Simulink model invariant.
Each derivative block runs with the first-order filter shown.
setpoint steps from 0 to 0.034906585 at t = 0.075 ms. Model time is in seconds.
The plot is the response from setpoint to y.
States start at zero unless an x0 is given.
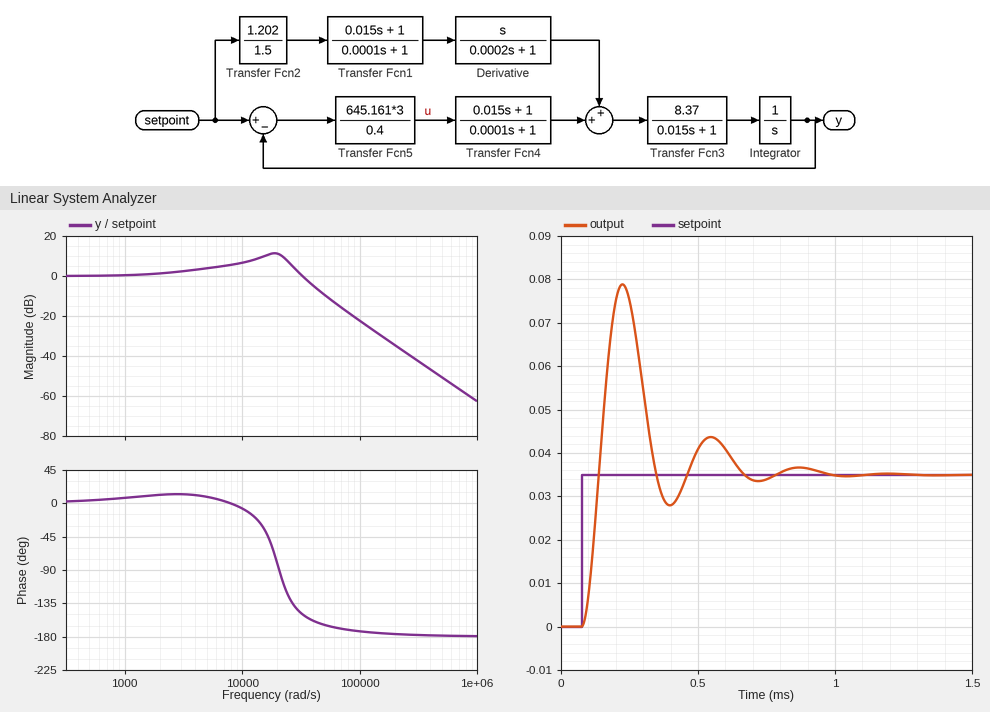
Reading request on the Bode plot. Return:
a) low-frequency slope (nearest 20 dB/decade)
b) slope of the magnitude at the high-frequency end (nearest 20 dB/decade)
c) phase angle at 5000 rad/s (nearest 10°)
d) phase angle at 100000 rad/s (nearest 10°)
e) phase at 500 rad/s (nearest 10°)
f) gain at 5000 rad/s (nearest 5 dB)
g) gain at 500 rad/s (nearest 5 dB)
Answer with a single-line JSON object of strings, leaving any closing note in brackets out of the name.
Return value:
{"low-frequency slope": "0 dB/decade", "slope of the magnitude at the high-frequency end": "-40 dB/decade", "phase angle at 5000 rad/s": "10°", "phase angle at 100000 rad/s": "-170°", "phase at 500 rad/s": "0°", "gain at 5000 rad/s": "5 dB", "gain at 500 rad/s": "0 dB"}
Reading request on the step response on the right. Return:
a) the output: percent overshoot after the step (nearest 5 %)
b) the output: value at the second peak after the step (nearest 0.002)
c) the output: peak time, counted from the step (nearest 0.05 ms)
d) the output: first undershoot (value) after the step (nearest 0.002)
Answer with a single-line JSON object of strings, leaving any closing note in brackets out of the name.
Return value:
{"the output: percent overshoot after the step": "125 %", "the output: value at the second peak after the step": "0.044", "the output: peak time, counted from the step": "0.15 ms", "the output: first undershoot (value) after the step": "0.028"}
